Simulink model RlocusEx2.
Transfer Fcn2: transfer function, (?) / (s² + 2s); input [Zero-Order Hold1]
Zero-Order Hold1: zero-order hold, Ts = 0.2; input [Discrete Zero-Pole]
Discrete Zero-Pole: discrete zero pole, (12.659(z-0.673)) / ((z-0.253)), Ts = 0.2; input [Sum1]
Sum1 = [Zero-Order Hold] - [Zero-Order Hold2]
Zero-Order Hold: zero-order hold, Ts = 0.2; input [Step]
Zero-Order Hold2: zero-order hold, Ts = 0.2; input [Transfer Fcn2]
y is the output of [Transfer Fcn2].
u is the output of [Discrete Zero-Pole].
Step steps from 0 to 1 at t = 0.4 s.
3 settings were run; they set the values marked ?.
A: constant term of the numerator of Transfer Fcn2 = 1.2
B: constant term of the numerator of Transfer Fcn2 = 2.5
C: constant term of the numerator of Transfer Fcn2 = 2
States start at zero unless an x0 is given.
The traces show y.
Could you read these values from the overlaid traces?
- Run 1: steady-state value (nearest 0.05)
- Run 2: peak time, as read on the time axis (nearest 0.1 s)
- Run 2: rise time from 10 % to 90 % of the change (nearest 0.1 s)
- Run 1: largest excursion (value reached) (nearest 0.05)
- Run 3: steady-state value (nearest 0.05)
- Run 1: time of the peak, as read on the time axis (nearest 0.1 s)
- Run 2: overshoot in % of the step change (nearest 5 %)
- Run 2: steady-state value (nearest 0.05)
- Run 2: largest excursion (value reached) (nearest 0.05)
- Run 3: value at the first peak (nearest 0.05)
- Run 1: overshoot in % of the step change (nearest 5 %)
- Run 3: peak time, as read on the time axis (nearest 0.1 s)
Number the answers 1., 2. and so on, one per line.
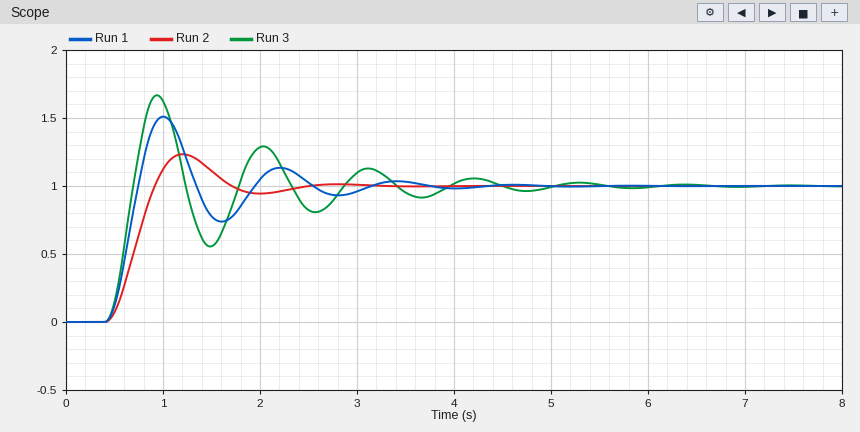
1. 1.00
2. 1.2 s
3. 0.3 s
4. 1.50
5. 1.00
6. 1.0 s
7. 25 %
8. 1.00
9. 1.25
10. 1.65
11. 50 %
12. 0.9 s
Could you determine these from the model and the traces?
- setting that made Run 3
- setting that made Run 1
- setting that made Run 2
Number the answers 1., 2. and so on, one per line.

1. B
2. C
3. A
